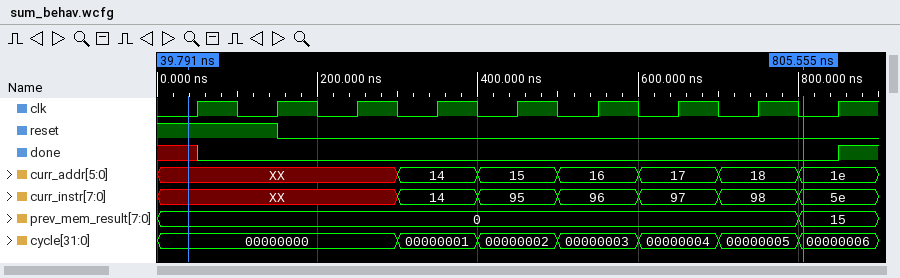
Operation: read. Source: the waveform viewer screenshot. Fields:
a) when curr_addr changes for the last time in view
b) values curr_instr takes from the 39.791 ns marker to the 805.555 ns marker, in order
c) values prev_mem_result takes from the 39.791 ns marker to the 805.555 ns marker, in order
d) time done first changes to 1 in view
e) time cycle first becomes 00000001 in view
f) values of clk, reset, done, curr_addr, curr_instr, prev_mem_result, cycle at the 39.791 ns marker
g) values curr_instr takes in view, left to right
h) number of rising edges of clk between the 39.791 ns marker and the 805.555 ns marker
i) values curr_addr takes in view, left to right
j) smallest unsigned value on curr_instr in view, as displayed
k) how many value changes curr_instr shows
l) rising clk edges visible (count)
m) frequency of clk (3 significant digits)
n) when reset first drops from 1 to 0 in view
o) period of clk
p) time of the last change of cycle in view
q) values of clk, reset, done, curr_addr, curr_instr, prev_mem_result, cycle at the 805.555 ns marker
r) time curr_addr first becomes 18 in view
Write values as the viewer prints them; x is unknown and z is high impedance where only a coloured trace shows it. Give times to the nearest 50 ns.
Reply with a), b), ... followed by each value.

a) 800 ns
b) XX, 14, 95, 96, 97, 98, 5e
c) 0, 15
d) 850 ns
e) 300 ns
f) clk=0, reset=1, done=x, curr_addr=XX, curr_instr=XX, prev_mem_result=0, cycle=00000000
g) XX, 14, 95, 96, 97, 98, 5e
h) 8
i) XX, 14, 15, 16, 17, 18, 1e
j) 14
k) 6
l) 9
m) 10.0 MHz
n) 150 ns
o) 100 ns
p) 800 ns
q) clk=0, reset=0, done=0, curr_addr=1e, curr_instr=5e, prev_mem_result=15, cycle=00000006
r) 700 ns
